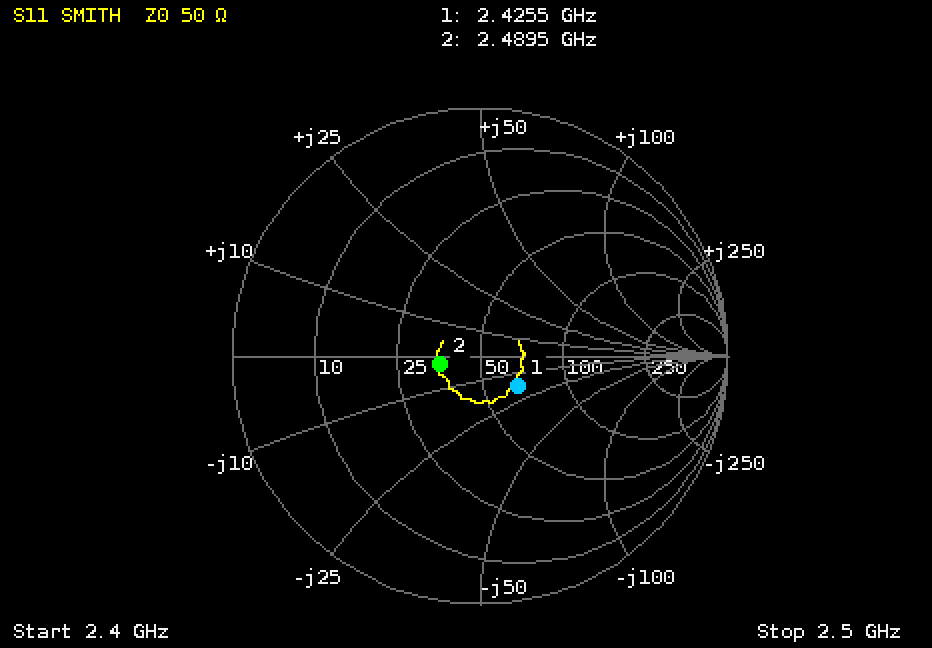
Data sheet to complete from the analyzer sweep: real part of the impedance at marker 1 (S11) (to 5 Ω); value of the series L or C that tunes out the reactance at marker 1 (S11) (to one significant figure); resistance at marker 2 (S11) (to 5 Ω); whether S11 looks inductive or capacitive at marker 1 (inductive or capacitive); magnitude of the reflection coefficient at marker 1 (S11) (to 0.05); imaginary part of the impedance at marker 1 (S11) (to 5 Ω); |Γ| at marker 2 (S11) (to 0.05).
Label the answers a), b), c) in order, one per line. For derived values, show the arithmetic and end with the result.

a) 65 Ω
b) L = 15 Ω/(2π × 2.4255 GHz) ≈ 1 nH
c) 35 Ω
d) capacitive
e) 0.20
f) -15 Ω
g) 0.15
